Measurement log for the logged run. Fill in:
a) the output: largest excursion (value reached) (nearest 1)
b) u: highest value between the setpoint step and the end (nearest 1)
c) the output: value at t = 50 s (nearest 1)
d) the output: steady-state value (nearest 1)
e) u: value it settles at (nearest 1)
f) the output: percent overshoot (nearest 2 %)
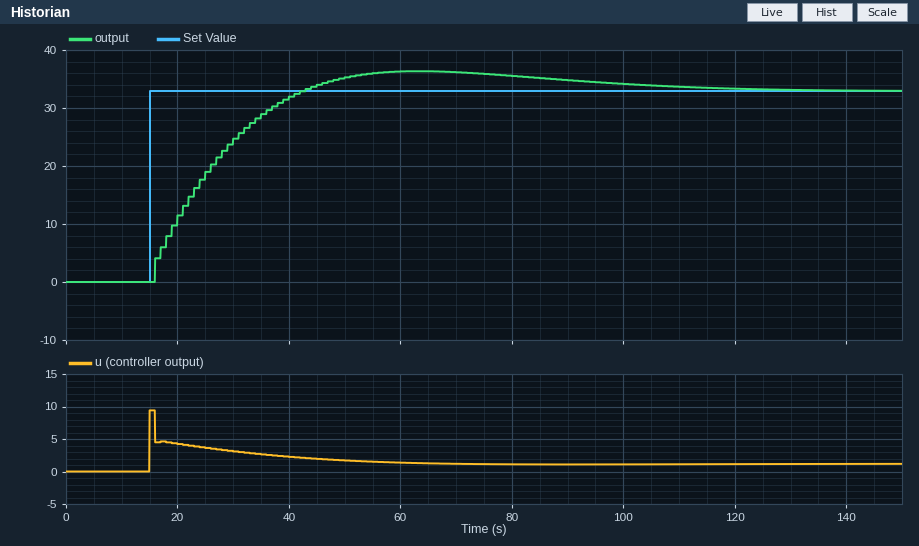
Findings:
36
9
35
33
1
10 %
